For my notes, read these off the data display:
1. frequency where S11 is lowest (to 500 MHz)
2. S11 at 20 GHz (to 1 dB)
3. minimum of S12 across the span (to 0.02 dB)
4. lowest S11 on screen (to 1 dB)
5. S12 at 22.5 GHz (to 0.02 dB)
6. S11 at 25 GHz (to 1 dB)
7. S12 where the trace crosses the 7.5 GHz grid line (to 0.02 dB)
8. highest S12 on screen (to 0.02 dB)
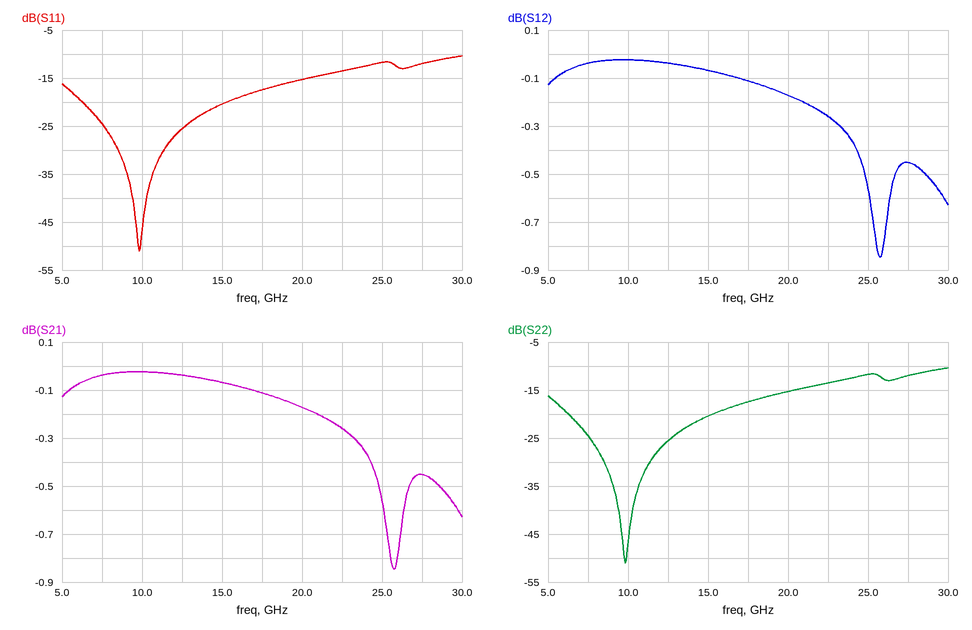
10.0 GHz
-15 dB
-0.84 dB
-51 dB
-0.26 dB
-12 dB
-0.04 dB
-0.02 dB
